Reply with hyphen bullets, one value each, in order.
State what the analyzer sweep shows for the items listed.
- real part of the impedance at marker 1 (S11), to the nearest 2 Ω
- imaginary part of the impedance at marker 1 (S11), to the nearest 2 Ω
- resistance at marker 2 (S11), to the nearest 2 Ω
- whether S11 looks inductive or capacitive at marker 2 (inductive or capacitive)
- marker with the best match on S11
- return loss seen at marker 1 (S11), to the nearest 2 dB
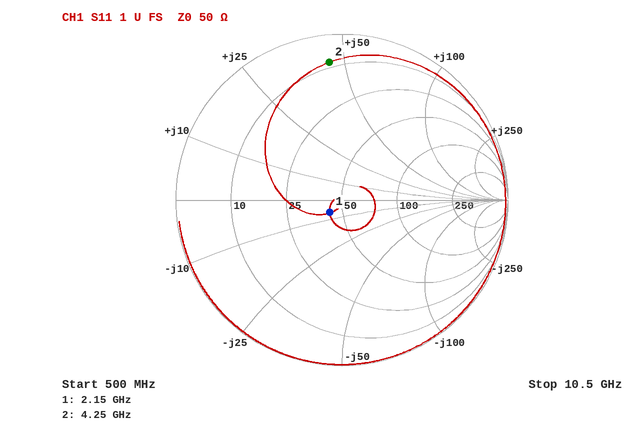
- 42 Ω
- -6 Ω
- 8 Ω
- inductive
- marker 1
- 20 dB
